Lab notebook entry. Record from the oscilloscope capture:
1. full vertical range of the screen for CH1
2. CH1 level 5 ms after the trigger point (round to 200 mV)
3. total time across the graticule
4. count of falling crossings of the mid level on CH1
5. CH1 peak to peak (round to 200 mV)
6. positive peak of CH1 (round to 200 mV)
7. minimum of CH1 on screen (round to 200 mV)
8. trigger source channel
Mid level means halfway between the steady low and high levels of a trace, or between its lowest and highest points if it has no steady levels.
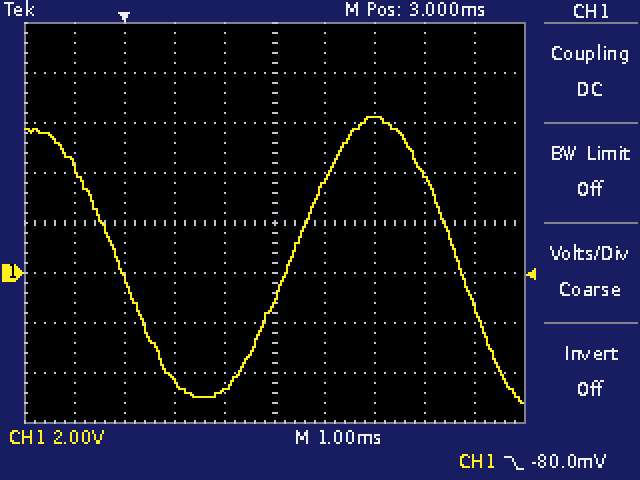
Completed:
16 V
6.2 V
10 ms
2
11.4 V
6.2 V
-5.2 V
CH1
